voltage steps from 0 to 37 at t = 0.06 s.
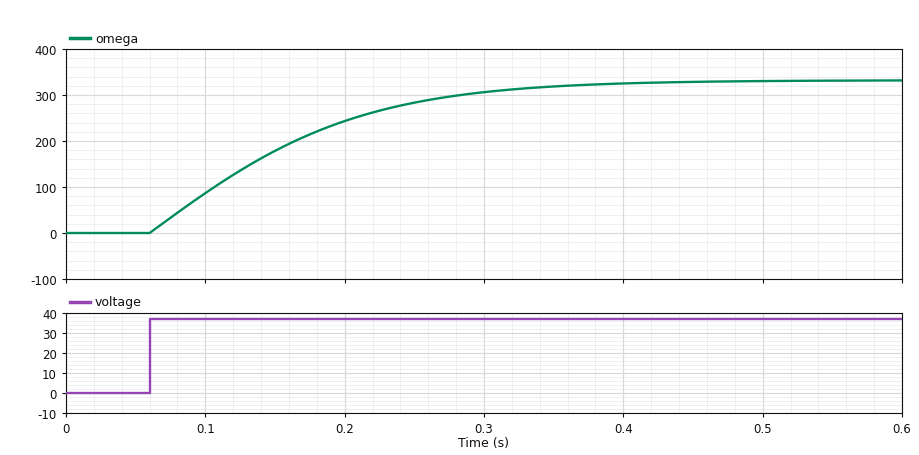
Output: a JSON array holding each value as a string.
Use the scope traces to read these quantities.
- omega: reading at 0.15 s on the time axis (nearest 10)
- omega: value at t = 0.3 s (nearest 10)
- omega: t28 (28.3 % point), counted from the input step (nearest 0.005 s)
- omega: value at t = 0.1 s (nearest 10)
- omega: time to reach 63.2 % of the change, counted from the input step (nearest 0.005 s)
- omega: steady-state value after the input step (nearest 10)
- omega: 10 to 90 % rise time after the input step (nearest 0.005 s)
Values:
["180", "310", "0.045 s", "90", "0.110 s", "330", "0.205 s"]
